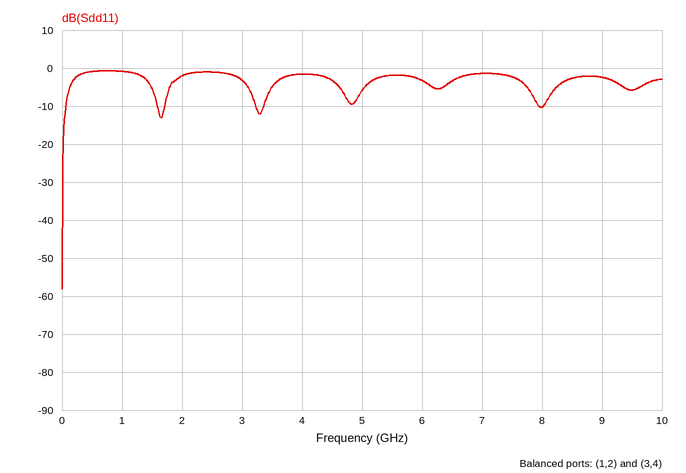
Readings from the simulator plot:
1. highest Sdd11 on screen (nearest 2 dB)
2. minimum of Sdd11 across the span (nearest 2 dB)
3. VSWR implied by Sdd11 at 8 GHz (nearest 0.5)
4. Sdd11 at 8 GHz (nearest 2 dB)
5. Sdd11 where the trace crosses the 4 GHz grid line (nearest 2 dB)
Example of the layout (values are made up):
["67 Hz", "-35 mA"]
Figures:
["0 dB", "-58 dB", "2.0", "-10 dB", "-2 dB"]
